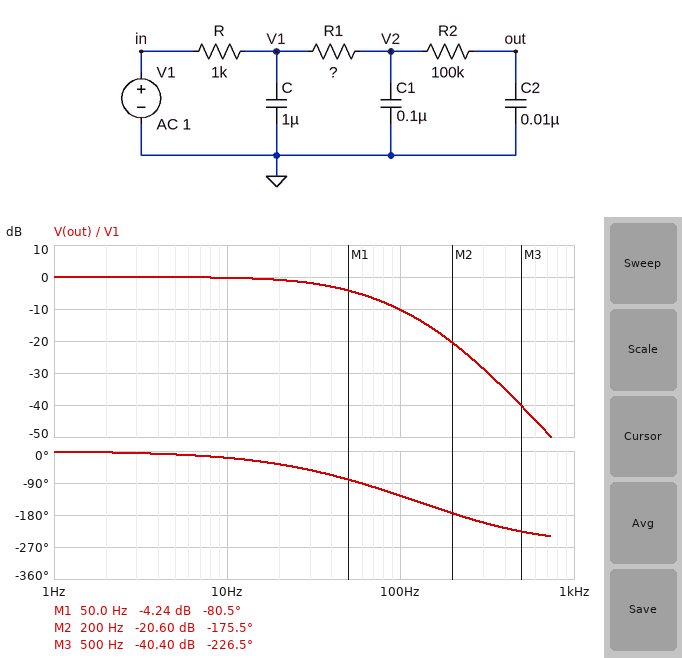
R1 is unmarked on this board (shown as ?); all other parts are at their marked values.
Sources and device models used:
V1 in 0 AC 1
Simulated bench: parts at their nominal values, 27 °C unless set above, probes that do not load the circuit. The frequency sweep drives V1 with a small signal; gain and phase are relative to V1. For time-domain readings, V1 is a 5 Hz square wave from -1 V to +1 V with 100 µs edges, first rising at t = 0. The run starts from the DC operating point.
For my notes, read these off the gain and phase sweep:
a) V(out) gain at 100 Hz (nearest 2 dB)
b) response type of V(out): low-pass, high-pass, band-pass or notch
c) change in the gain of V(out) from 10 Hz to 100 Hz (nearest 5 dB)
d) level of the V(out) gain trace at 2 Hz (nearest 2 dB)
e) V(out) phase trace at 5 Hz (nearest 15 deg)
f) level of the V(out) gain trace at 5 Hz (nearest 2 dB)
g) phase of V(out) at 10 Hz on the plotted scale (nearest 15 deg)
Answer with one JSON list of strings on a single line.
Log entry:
["-10 dB", "low-pass", "-10 dB", "0 dB", "-15 deg", "0 dB", "-15 deg"]
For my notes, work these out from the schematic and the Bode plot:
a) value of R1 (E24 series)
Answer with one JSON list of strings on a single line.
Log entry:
["30 kΩ"]
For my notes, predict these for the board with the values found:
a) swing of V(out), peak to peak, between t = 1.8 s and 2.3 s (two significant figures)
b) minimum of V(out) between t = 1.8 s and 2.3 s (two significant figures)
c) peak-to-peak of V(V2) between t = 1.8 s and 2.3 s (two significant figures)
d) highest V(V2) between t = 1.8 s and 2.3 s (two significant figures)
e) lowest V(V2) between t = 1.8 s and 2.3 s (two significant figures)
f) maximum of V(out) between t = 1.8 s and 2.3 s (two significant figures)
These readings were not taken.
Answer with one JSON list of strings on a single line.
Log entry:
["2.0 V", "-1.0 V", "2.0 V", "1.0 V", "-1.0 V", "1.0 V"]
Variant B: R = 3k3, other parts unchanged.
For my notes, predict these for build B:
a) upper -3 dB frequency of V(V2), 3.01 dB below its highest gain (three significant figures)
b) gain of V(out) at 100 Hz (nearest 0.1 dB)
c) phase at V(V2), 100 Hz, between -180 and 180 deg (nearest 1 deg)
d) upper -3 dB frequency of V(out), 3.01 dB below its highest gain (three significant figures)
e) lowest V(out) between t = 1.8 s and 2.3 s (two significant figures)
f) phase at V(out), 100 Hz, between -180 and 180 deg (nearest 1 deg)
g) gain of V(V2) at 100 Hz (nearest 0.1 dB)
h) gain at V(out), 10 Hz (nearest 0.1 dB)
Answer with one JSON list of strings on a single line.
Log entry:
["28.5 Hz", "-16.2 dB", "-125 deg", "27.7 Hz", "-1.0 V", "-157 deg", "-14.7 dB", "-0.5 dB"]
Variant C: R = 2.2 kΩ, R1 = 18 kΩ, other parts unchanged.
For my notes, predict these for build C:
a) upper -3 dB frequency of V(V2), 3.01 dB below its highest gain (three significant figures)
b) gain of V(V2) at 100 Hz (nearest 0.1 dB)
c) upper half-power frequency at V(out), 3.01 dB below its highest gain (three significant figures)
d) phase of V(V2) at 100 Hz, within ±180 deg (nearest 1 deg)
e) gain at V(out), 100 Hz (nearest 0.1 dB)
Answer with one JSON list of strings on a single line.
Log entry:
["44.6 Hz", "-9.2 dB", "41.9 Hz", "-102 deg", "-10.6 dB"]
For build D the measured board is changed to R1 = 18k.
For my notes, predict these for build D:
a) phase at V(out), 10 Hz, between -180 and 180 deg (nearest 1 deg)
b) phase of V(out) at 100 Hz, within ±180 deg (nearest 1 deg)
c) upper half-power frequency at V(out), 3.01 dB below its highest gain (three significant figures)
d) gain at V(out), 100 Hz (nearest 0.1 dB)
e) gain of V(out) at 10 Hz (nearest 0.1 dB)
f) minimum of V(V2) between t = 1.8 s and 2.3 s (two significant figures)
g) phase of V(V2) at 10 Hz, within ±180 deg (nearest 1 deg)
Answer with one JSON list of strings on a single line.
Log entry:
["-15 deg", "-114 deg", "55.8 Hz", "-7.3 dB", "-0.1 dB", "-1.0 V", "-11 deg"]
